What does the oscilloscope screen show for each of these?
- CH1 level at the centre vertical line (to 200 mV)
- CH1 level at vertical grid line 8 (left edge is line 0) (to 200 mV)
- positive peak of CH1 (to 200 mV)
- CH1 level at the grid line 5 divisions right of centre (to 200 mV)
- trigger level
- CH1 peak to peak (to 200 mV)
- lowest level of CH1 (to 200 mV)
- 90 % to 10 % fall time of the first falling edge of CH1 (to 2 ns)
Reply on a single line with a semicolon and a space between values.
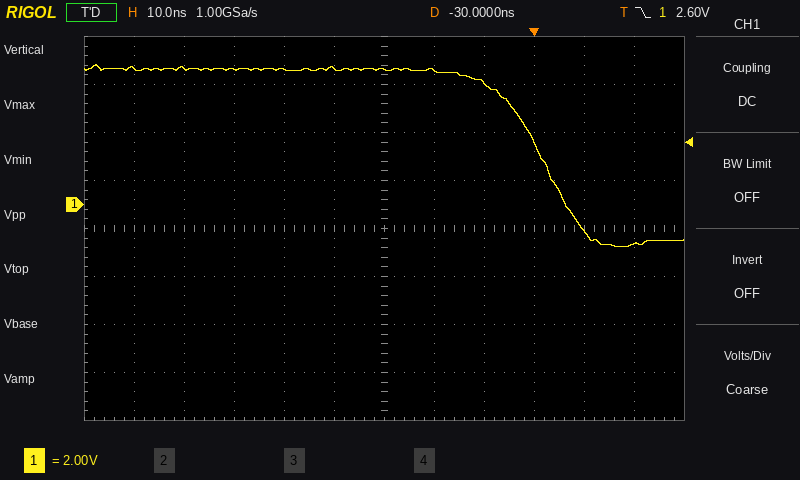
5.6 V; 5.0 V; 5.8 V; -1.6 V; 2.60 V; 7.6 V; -1.8 V; 18 ns
